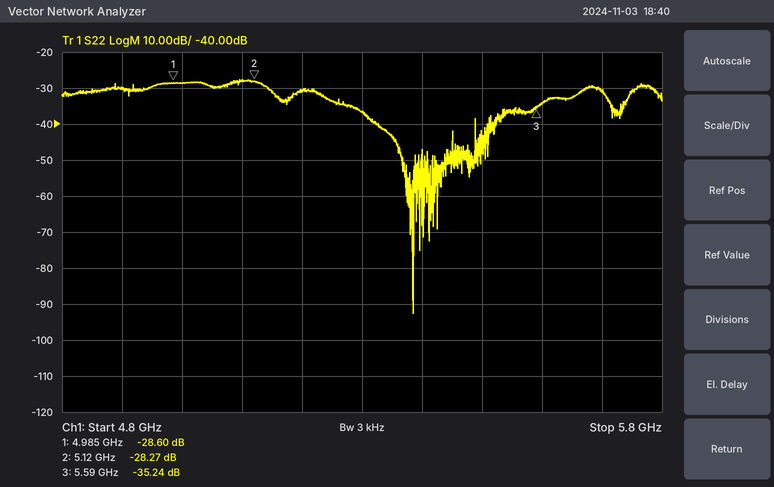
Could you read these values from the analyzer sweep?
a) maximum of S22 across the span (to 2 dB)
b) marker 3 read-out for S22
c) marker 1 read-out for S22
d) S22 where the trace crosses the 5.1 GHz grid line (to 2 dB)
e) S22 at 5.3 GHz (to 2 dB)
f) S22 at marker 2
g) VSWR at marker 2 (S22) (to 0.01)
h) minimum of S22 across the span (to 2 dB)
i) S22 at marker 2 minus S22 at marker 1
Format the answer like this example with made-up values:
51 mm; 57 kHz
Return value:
-28 dB; -35.24 dB; -28.60 dB; -28 dB; -36 dB; -28.27 dB; 1.08; -92 dB; 0.33 dB
